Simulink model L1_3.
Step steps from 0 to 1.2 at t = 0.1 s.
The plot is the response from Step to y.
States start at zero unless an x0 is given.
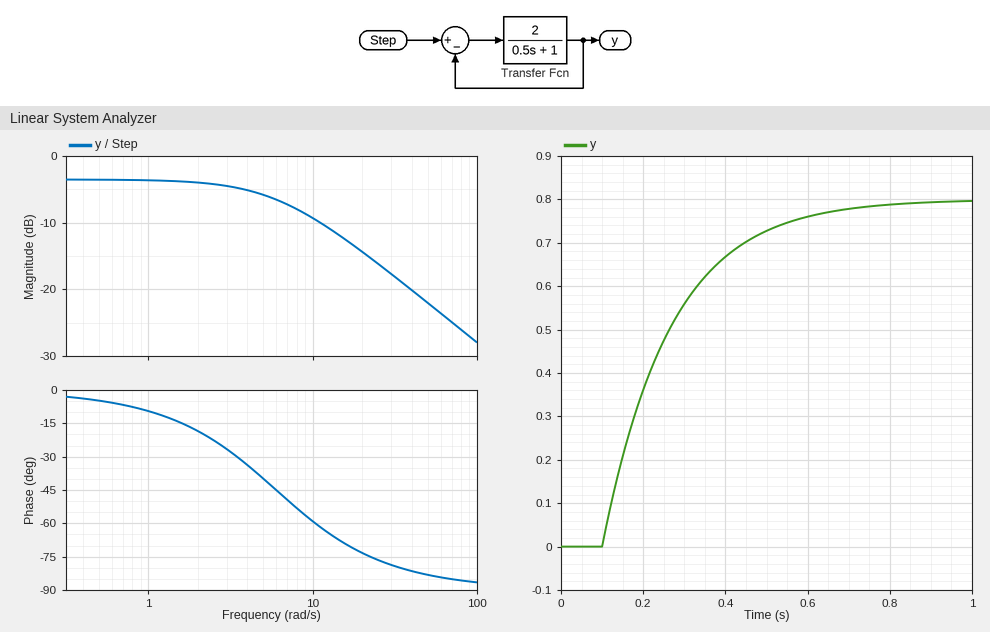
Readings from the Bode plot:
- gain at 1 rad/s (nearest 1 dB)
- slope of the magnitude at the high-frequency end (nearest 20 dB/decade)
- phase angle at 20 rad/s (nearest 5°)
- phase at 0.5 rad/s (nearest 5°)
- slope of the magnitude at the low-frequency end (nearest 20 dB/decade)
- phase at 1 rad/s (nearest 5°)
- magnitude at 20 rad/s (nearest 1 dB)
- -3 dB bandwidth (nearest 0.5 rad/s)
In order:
-4 dB
-20 dB/decade
-75°
-5°
0 dB/decade
-10°
-14 dB
6.0 rad/s
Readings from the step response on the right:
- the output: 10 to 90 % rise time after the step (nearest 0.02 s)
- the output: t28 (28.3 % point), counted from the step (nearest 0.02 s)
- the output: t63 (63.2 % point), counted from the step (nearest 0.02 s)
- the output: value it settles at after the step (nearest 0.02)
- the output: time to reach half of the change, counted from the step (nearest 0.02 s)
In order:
0.36 s
0.06 s
0.16 s
0.80
0.12 s
